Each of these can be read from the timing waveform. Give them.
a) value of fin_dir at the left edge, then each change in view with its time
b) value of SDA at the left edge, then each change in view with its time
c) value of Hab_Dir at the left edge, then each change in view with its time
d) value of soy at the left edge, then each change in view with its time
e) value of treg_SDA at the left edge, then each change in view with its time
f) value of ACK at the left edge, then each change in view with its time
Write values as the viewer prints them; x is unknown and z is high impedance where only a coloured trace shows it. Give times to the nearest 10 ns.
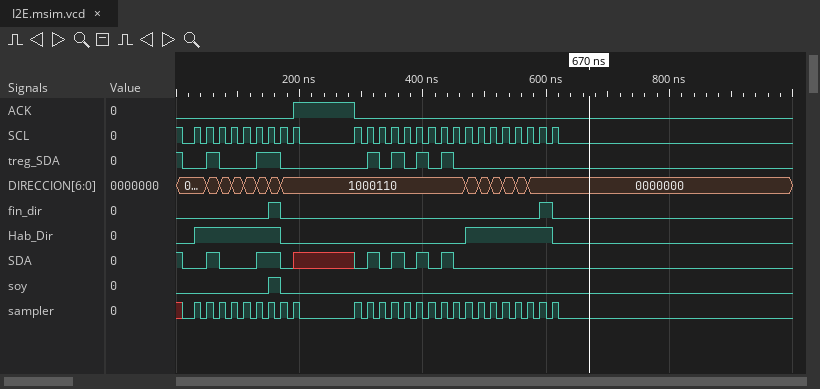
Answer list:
0, 1 at 150 ns, 0 at 170 ns, 1 at 590 ns, 0 at 610 ns
1, 0 at 10 ns, 1 at 50 ns, 0 at 70 ns, 1 at 130 ns, 0 at 170 ns, x at 190 ns, 0 at 290 ns, 1 at 310 ns, 0 at 330 ns, 1 at 350 ns, 0 at 370 ns, 1 at 390 ns, 0 at 410 ns, 1 at 430 ns, 0 at 450 ns
0, 1 at 30 ns, 0 at 170 ns, 1 at 470 ns, 0 at 610 ns
0, 1 at 150 ns, 0 at 170 ns
1, 0 at 10 ns, 1 at 50 ns, 0 at 70 ns, 1 at 130 ns, 0 at 170 ns, 1 at 310 ns, 0 at 330 ns, 1 at 350 ns, 0 at 370 ns, 1 at 390 ns, 0 at 410 ns, 1 at 430 ns, 0 at 450 ns
0, 1 at 190 ns, 0 at 290 ns
